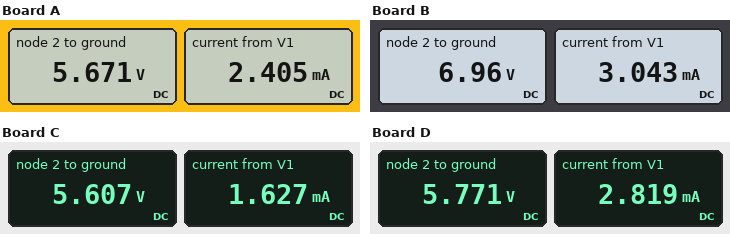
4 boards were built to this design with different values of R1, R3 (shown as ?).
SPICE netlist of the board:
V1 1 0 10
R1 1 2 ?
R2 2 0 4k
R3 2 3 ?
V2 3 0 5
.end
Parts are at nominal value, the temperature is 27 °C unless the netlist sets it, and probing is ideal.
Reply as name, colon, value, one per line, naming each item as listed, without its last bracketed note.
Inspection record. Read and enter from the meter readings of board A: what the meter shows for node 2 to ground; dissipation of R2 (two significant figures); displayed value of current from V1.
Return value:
what the meter shows for node 2 to ground: 5.671 V
dissipation of R2: 8.0 mW
displayed value of current from V1: 2.405 mA
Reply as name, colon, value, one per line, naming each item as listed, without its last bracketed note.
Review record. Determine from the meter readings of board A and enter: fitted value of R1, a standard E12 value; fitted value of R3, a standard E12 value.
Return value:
fitted value of R1, a standard E12 value: 1.8 kΩ
fitted value of R3, a standard E12 value: 680 Ω
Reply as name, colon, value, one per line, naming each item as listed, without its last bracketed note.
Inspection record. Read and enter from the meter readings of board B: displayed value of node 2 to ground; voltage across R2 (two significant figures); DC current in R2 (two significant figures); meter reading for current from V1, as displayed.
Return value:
displayed value of node 2 to ground: 6.96 V
voltage across R2: 7.0 V
DC current in R2: 1.7 mA
meter reading for current from V1, as displayed: 3.043 mA
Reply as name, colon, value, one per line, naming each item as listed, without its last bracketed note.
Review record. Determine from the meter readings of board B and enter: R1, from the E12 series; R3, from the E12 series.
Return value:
R1, from the E12 series: 1 kΩ
R3, from the E12 series: 1.5 kΩ
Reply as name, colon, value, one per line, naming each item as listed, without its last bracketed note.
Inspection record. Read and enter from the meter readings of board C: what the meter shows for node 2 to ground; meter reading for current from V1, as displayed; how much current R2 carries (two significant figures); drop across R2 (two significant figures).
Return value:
what the meter shows for node 2 to ground: 5.607 V
meter reading for current from V1, as displayed: 1.627 mA
how much current R2 carries: 1.4 mA
drop across R2: 5.6 V
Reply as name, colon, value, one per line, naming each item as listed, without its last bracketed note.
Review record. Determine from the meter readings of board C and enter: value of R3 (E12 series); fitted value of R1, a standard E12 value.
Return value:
value of R3: 2.7 kΩ
fitted value of R1, a standard E12 value: 2.7 kΩ
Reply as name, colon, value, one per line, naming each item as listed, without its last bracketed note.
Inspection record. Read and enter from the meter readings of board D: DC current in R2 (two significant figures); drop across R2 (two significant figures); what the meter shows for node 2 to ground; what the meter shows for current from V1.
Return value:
DC current in R2: 1.4 mA
drop across R2: 5.8 V
what the meter shows for node 2 to ground: 5.771 V
what the meter shows for current from V1: 2.819 mA
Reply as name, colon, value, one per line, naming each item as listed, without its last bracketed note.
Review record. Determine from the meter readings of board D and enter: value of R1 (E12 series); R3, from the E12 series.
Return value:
value of R1: 1.5 kΩ
R3, from the E12 series: 560 Ω
